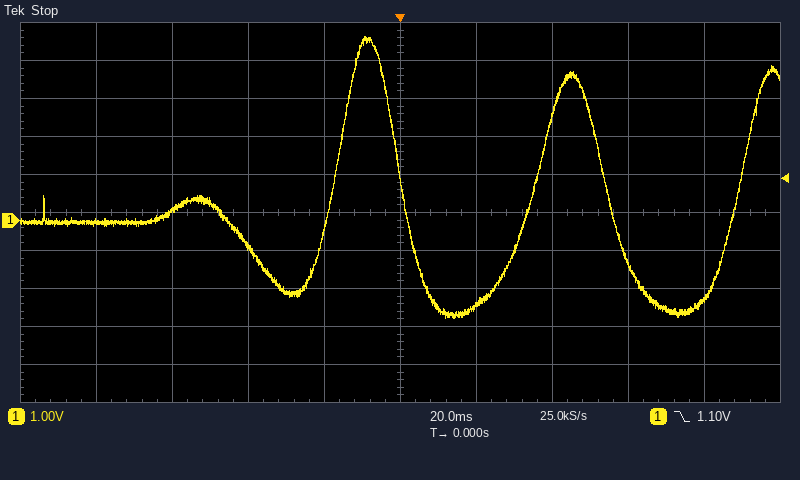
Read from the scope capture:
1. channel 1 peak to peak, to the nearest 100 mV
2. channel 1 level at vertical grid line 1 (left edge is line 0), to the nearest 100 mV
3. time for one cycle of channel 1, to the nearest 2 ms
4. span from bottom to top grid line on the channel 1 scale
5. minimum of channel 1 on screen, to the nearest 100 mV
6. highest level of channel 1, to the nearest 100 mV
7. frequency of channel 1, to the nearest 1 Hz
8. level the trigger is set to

7.4 V
-100 mV
54 ms
10 V
-2.6 V
4.8 V
19 Hz
1.10 V
